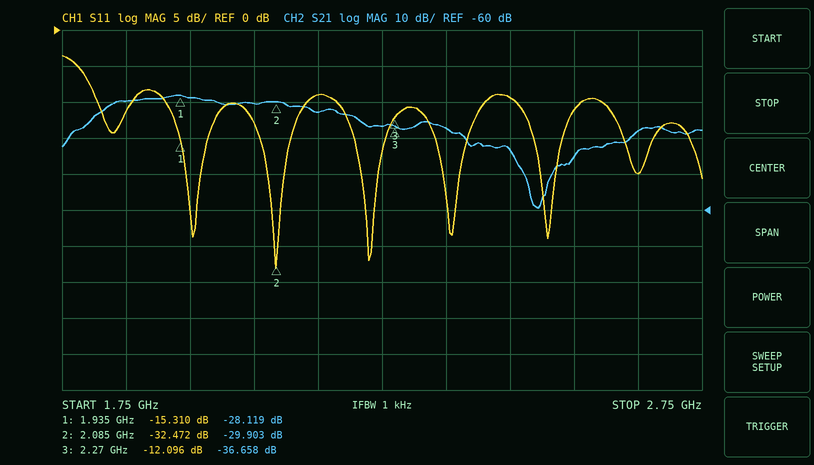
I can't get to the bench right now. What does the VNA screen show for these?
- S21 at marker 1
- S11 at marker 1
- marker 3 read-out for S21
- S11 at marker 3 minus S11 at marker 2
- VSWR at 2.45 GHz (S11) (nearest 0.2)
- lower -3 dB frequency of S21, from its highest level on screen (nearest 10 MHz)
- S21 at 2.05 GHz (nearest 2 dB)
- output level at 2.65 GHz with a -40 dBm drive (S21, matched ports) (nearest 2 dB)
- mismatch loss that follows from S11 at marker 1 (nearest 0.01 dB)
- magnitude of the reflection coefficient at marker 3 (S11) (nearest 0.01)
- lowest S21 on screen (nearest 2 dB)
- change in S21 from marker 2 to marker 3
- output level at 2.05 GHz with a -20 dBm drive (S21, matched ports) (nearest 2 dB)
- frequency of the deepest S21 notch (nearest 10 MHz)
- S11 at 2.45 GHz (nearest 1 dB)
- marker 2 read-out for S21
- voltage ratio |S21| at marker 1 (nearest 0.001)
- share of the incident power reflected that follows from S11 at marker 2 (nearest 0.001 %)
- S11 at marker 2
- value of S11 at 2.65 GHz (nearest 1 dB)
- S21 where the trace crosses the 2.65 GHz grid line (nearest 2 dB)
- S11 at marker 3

-28.119 dB
-15.310 dB
-36.658 dB
20.376 dB
2.0
1.82 GHz
-30 dB
-78 dBm
0.13 dB
0.25
-60 dB
-6.755 dB
-50 dBm
2.49 GHz
-9 dB
-29.903 dB
0.039
0.057 %
-32.472 dB
-20 dB
-38 dB
-12.096 dB
